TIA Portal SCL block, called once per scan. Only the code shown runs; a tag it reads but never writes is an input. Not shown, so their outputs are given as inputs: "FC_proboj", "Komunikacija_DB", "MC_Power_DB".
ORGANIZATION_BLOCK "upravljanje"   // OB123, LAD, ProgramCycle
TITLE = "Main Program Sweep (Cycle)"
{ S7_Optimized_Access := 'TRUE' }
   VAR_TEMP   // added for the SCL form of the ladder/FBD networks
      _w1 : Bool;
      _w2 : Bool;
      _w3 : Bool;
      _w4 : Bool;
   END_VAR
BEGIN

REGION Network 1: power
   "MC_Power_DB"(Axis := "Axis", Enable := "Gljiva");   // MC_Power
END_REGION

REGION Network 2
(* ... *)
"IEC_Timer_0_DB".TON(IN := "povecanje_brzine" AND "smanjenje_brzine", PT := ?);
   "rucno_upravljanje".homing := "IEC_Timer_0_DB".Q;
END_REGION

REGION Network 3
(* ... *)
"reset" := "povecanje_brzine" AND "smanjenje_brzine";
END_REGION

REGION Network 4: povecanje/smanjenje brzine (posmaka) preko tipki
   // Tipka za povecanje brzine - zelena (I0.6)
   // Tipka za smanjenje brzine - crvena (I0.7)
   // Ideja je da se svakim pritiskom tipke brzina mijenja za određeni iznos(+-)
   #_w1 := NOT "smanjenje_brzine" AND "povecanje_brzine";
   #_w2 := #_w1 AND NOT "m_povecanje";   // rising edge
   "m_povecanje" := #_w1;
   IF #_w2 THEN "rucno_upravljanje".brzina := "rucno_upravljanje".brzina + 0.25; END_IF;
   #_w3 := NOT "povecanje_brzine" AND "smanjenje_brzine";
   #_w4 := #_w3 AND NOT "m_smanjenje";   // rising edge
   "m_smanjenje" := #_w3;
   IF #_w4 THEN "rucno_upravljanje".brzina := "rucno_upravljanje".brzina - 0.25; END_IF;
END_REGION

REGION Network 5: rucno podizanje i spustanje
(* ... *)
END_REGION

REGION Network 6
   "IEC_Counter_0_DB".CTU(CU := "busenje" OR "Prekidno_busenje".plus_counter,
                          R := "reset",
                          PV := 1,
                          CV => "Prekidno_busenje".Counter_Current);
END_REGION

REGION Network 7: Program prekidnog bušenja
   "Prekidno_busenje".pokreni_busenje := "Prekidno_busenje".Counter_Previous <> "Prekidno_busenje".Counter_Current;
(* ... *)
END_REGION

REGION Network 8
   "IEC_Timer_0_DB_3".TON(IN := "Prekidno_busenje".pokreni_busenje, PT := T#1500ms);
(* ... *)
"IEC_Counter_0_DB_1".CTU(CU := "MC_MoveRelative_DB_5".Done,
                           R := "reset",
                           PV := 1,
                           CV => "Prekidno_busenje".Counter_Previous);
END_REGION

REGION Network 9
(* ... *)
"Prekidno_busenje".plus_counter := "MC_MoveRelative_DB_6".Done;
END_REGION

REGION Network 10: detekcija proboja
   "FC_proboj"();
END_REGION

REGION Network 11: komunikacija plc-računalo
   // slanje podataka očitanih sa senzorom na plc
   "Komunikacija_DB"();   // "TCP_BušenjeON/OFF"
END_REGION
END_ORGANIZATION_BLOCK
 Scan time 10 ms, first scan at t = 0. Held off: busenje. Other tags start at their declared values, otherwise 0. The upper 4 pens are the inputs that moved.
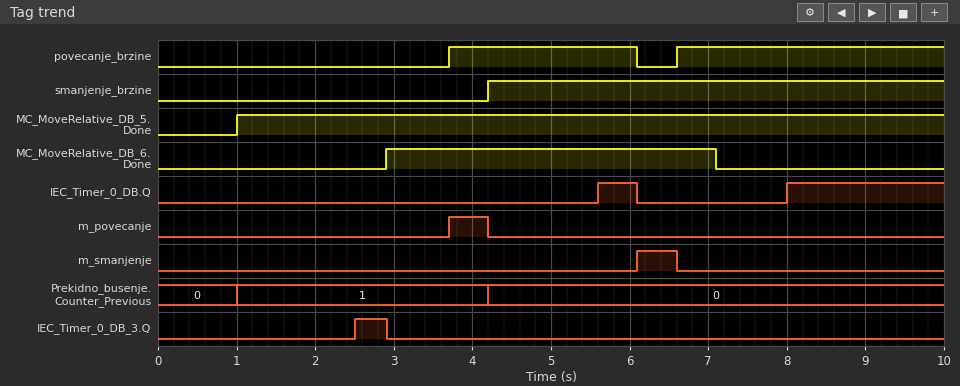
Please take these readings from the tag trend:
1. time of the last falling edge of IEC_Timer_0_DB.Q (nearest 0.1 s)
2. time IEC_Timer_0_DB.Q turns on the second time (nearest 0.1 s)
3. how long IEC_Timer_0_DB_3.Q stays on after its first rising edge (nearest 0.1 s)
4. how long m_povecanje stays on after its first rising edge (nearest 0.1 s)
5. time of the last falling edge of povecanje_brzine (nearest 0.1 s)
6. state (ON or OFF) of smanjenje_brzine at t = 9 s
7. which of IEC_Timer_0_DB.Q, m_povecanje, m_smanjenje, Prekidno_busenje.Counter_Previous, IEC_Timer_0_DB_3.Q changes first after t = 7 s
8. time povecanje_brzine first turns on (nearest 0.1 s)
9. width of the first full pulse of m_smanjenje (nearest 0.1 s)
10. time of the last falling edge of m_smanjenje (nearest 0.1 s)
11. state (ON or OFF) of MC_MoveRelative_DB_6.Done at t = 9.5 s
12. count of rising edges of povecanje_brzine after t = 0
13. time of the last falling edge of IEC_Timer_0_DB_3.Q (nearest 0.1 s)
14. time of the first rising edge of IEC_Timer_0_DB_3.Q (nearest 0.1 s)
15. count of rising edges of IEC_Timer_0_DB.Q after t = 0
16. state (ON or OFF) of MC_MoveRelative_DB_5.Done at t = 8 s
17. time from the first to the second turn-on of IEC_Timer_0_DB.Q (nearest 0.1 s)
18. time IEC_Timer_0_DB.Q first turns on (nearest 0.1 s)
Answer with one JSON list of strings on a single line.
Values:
["6.1 s", "8.0 s", "0.4 s", "0.5 s", "6.1 s", "ON", "IEC_Timer_0_DB.Q", "3.7 s", "0.5 s", "6.6 s", "OFF", "2", "2.9 s", "2.5 s", "2", "ON", "2.4 s", "5.6 s"]
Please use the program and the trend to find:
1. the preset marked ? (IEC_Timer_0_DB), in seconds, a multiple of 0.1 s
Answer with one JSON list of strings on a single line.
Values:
["1.4 s"]
